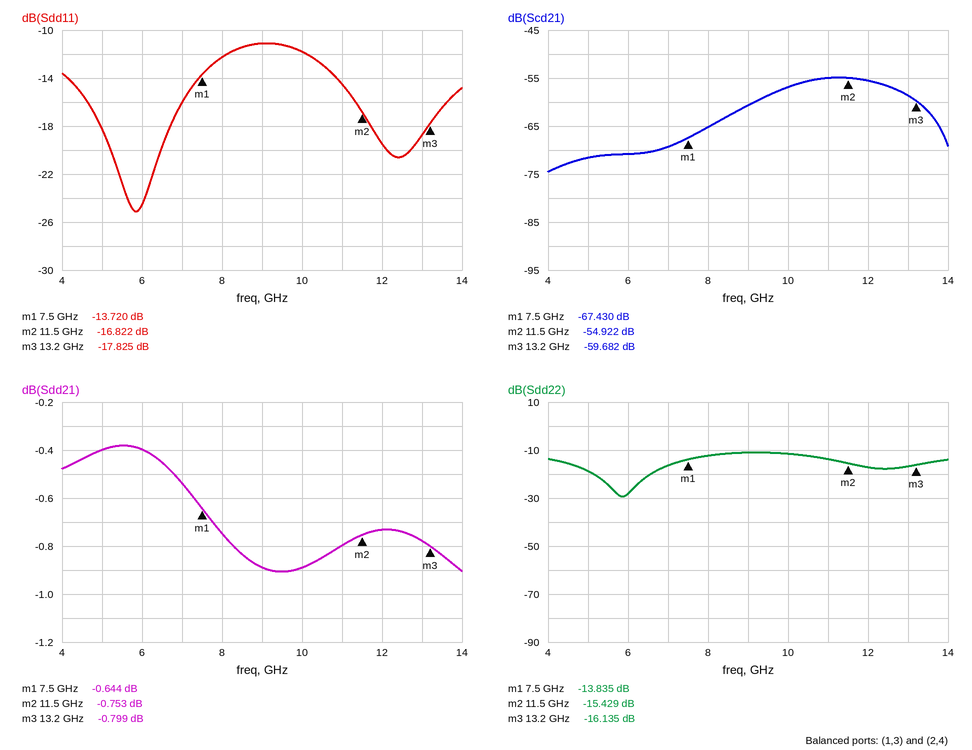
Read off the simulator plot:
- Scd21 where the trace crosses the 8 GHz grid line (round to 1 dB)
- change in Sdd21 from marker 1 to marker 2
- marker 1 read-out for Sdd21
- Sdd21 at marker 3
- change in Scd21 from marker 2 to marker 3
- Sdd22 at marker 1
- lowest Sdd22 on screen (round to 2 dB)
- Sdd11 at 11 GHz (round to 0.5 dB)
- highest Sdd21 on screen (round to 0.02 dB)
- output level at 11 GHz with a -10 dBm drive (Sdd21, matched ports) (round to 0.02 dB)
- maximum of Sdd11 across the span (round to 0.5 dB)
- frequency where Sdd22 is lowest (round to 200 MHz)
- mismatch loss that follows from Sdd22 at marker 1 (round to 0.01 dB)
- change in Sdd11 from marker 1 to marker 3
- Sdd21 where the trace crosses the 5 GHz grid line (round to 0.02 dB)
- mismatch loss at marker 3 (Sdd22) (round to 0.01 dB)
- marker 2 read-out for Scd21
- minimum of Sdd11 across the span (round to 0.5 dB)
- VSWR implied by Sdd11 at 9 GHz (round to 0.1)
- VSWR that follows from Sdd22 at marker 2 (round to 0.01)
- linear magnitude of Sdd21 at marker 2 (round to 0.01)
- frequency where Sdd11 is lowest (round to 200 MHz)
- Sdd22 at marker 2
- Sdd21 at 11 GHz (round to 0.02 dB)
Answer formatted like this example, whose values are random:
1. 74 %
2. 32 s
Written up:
1. -65 dB
2. -0.109 dB
3. -0.644 dB
4. -0.799 dB
5. -4.760 dB
6. -13.835 dB
7. -30 dB
8. -14.5 dB
9. -0.38 dB
10. -10.80 dBm
11. -11.0 dB
12. 5.8 GHz
13. 0.18 dB
14. -4.105 dB
15. -0.40 dB
16. 0.11 dB
17. -54.922 dB
18. -25.0 dB
19. 1.8
20. 1.41
21. 0.92
22. 5.8 GHz
23. -15.429 dB
24. -0.80 dB
